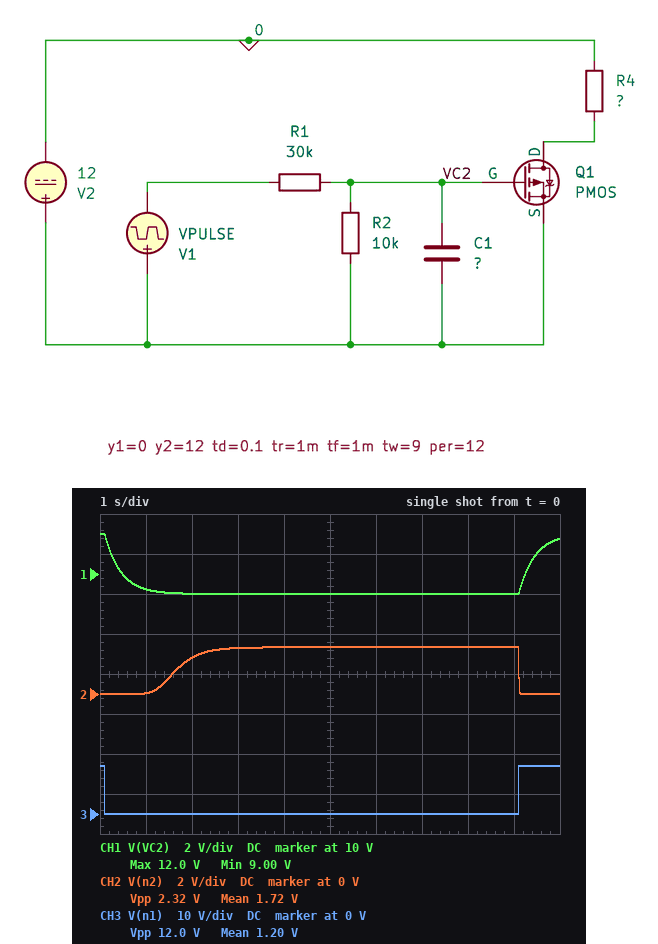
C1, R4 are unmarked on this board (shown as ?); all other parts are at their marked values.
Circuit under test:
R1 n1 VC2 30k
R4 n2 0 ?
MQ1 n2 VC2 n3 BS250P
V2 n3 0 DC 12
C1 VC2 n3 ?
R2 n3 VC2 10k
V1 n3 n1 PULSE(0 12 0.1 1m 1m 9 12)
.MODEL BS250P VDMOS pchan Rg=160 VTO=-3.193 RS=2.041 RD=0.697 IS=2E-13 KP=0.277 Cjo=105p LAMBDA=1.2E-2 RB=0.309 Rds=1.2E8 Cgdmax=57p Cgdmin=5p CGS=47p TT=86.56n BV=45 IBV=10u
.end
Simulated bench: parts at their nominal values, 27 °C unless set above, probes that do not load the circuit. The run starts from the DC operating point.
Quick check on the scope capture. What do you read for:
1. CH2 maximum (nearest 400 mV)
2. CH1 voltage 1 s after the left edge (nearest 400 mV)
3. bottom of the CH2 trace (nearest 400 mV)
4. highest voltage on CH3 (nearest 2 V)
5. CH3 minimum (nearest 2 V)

2.4 V
9.2 V
0 V
12 V
0 V
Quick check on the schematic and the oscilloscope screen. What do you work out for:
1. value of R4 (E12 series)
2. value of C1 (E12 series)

82 kΩ
47 µF
